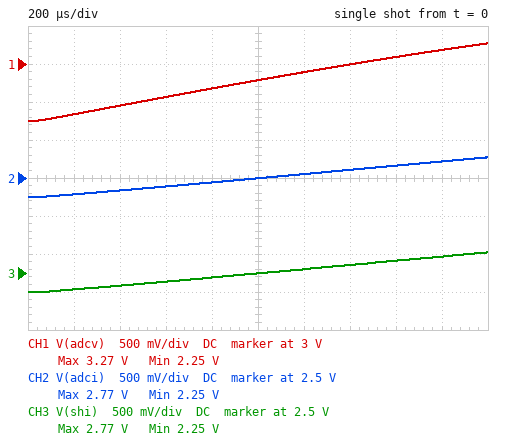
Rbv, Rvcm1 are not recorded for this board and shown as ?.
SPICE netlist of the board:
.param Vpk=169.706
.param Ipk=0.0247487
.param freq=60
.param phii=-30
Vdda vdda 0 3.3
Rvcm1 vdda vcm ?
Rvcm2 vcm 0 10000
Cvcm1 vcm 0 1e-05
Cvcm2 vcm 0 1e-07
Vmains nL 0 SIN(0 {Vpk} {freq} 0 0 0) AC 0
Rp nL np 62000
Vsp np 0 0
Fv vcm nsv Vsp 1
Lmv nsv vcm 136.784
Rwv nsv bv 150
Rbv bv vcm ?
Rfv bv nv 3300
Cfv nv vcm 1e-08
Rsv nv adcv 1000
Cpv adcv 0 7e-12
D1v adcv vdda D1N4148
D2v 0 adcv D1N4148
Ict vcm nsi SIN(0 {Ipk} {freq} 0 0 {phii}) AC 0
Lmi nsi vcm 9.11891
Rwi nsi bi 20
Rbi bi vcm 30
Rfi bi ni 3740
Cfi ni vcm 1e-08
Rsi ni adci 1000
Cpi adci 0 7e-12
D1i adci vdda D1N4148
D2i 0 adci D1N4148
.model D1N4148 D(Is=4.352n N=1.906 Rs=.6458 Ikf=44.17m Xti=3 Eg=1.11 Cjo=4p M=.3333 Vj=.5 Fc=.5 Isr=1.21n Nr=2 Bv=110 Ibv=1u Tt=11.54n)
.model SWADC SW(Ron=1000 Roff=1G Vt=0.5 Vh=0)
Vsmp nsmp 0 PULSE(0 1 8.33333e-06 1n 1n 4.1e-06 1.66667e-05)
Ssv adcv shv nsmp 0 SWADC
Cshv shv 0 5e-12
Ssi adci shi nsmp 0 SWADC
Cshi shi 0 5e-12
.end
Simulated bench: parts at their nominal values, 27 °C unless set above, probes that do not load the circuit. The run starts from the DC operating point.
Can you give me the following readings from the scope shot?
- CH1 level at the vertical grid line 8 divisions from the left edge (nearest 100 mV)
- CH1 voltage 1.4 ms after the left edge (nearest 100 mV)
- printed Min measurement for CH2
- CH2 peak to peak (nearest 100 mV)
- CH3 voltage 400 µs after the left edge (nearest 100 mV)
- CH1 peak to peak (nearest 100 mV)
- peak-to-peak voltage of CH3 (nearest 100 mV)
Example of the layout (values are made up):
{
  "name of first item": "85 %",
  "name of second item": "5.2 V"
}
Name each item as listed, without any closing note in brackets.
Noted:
{
  "CH1 level at the vertical grid line 8 divisions from the left edge": "3.1 V",
  "CH1 voltage 1.4 ms after the left edge": "3.0 V",
  "printed Min measurement for CH2": "2.25 V",
  "CH2 peak to peak": "500 mV",
  "CH3 voltage 400 µs after the left edge": "2.3 V",
  "CH1 peak to peak": "1.0 V",
  "peak-to-peak voltage of CH3": "500 mV"
}
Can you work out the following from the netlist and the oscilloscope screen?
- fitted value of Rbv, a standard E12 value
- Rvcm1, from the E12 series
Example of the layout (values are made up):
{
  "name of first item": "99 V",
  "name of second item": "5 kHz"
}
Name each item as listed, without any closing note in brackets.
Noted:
{
  "fitted value of Rbv, a standard E12 value": "560 Ω",
  "Rvcm1, from the E12 series": "4.7 kΩ"
}
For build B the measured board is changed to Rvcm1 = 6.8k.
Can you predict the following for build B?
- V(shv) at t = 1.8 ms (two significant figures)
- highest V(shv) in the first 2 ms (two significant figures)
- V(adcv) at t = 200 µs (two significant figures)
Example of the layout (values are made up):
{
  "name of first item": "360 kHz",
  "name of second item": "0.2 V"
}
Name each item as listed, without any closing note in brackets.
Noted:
{
  "V(shv) at t = 1.8 ms": "2.9 V",
  "highest V(shv) in the first 2 ms": "3.0 V",
  "V(adcv) at t = 200 µs": "2.1 V"
}
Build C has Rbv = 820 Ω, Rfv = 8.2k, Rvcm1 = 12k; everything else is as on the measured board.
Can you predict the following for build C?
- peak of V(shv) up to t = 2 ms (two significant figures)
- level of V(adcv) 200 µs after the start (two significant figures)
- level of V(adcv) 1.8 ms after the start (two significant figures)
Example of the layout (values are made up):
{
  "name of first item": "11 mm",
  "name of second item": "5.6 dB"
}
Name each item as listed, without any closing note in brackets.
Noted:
{
  "peak of V(shv) up to t = 2 ms": "3.0 V",
  "level of V(adcv) 200 µs after the start": "1.6 V",
  "level of V(adcv) 1.8 ms after the start": "2.8 V"
}
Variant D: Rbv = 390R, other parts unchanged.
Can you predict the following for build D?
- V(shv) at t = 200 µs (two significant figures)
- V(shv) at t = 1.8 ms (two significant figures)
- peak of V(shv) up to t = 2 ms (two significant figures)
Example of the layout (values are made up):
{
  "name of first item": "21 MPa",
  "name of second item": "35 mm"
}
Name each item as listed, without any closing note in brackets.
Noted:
{
  "V(shv) at t = 200 µs": "2.3 V",
  "V(shv) at t = 1.8 ms": "2.9 V",
  "peak of V(shv) up to t = 2 ms": "3.0 V"
}
